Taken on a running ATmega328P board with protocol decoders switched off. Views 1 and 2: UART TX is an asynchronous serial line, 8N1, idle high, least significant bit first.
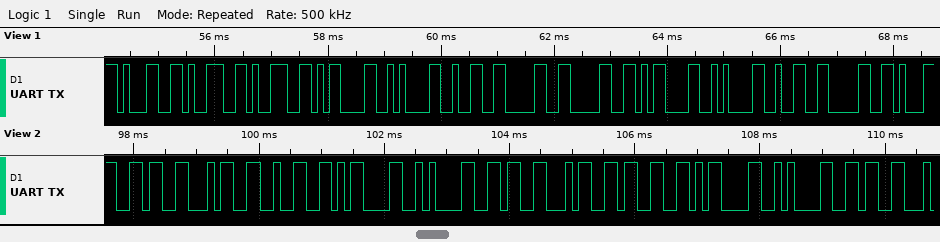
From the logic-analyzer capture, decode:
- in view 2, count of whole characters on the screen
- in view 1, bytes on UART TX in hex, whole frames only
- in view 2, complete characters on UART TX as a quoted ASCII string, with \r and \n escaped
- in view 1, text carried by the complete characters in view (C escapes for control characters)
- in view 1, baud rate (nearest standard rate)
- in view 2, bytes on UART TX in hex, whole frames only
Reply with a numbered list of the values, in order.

1. 11
2. 31 39 39 0D 0A 32 30 30 0D 0A 32 30
3. "642\r\n643\r\n6"
4. "199\r\n200\r\n20"
5. 9600 baud
6. 36 34 32 0D 0A 36 34 33 0D 0A 36
